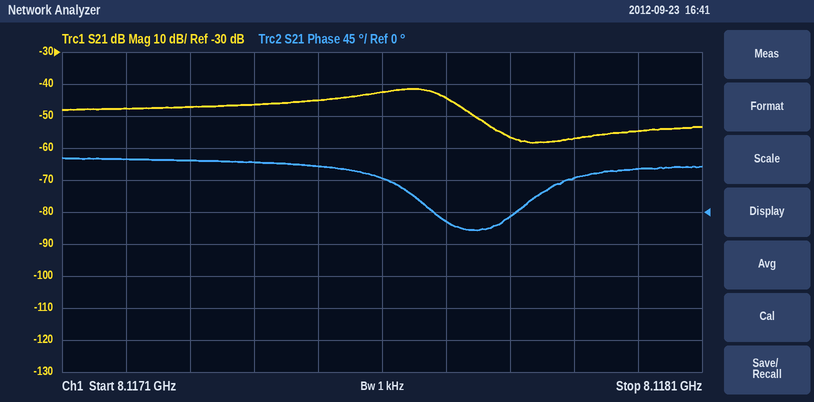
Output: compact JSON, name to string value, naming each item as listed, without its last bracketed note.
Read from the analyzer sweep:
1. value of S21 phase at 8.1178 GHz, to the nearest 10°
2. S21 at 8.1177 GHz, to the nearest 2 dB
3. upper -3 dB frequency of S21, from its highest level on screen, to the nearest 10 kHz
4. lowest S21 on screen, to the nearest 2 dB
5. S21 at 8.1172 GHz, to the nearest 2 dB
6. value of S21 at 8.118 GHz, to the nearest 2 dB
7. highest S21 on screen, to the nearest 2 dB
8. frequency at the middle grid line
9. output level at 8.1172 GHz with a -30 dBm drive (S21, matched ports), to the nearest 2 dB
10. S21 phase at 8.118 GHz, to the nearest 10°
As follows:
{"value of S21 phase at 8.1178 GHz, to the nearest 10°": "-10°", "S21 at 8.1177 GHz, to the nearest 2 dB": "-44 dB", "upper -3 dB frequency of S21, from its highest level on screen, to the nearest 10 kHz": "8.11770 GHz", "lowest S21 on screen, to the nearest 2 dB": "-58 dB", "S21 at 8.1172 GHz, to the nearest 2 dB": "-48 dB", "value of S21 at 8.118 GHz, to the nearest 2 dB": "-54 dB", "highest S21 on screen, to the nearest 2 dB": "-42 dB", "frequency at the middle grid line": "8.1176 GHz", "output level at 8.1172 GHz with a -30 dBm drive (S21, matched ports), to the nearest 2 dB": "-78 dBm", "S21 phase at 8.118 GHz, to the nearest 10°": "60°"}
